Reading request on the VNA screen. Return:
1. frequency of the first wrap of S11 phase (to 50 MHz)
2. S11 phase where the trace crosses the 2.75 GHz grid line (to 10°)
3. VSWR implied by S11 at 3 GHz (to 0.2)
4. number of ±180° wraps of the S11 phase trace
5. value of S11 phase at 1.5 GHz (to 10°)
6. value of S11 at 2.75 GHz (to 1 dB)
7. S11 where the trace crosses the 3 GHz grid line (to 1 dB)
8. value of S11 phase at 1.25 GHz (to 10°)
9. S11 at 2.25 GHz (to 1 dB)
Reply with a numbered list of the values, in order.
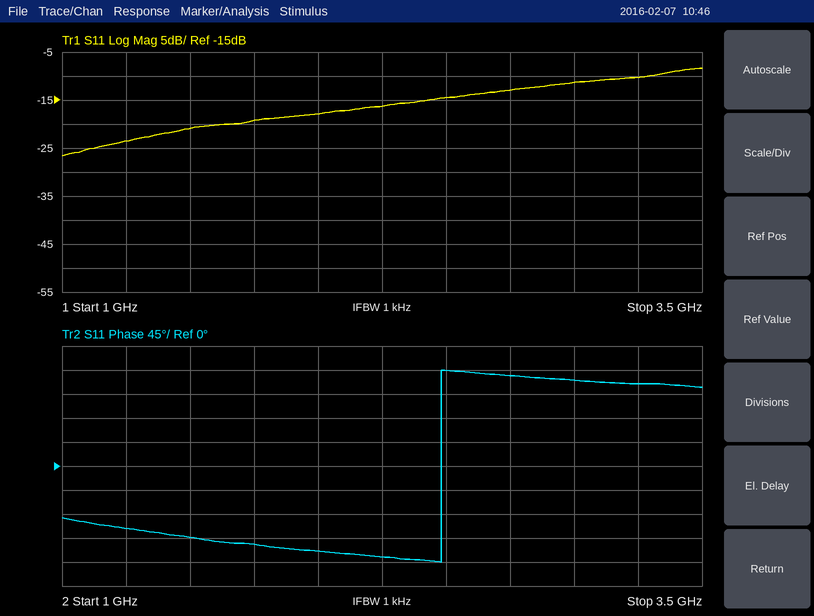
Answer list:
1. 2.50 GHz
2. 170°
3. 1.8
4. 1
5. -130°
6. -13 dB
7. -11 dB
8. -120°
9. -16 dB
